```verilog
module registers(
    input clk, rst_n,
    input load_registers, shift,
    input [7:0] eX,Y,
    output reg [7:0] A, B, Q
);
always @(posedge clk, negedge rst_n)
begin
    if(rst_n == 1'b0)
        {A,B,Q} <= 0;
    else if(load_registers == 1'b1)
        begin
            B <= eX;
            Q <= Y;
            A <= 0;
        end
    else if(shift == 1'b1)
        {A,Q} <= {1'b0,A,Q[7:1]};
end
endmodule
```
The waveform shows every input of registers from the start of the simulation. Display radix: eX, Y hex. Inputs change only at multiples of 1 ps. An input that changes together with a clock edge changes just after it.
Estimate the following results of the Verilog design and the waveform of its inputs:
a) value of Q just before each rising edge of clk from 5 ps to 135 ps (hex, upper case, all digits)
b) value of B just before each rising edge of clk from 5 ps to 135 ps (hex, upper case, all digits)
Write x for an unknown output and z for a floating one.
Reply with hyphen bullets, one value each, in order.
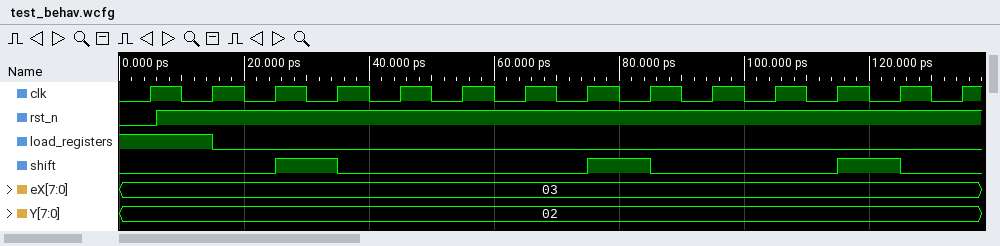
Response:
- 00, 00, 02, 02, 01, 01, 01, 01, 01, 00, 00, 00, 00, 00
- 00, 00, 03, 03, 03, 03, 03, 03, 03, 03, 03, 03, 03, 03
